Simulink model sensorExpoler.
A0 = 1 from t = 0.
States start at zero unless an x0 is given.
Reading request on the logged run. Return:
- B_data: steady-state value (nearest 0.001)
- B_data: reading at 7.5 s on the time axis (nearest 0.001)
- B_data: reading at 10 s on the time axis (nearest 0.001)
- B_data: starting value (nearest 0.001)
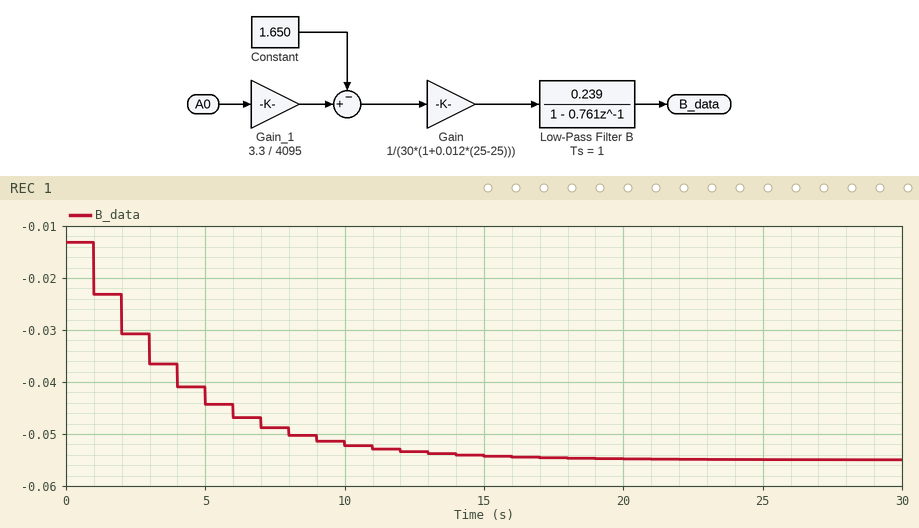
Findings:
-0.055
-0.049
-0.052
-0.013
